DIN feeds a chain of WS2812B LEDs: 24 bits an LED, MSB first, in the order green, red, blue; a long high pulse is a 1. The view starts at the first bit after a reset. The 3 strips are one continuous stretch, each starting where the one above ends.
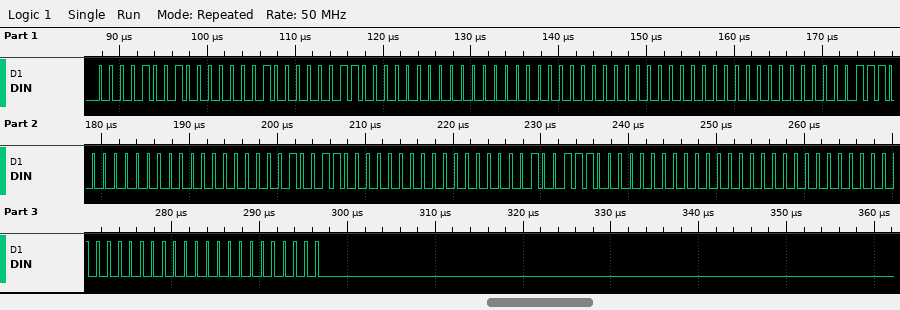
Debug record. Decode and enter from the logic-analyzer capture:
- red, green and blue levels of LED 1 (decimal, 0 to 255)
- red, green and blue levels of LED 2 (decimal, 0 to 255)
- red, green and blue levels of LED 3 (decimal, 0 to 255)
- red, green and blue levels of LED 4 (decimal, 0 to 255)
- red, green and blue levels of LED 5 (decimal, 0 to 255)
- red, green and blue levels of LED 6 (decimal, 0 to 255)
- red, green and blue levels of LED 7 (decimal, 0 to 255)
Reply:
1, 9, 3
0, 0, 0
0, 0, 7
0, 0, 19
0, 0, 78
0, 0, 0
0, 0, 0
